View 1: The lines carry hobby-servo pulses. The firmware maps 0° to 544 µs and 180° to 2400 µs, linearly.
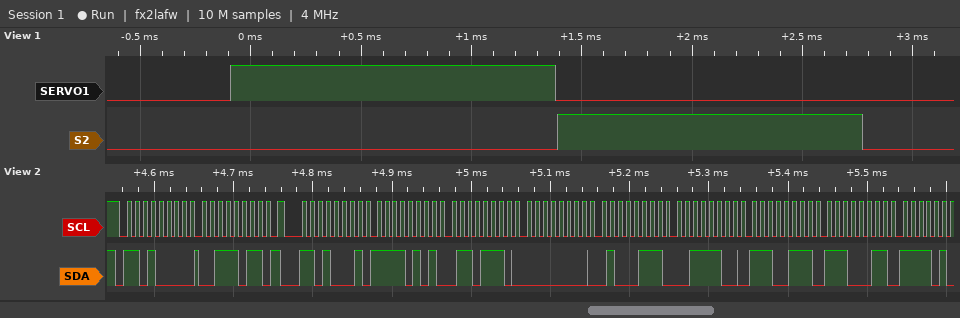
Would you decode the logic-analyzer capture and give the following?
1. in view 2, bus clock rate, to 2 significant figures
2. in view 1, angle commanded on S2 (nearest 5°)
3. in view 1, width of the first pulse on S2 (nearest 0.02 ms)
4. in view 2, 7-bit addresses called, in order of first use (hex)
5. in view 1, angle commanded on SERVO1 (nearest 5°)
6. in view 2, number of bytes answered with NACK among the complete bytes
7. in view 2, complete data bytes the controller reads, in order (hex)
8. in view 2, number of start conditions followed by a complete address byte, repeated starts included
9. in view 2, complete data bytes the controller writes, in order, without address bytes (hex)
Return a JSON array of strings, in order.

["100 kHz", "80°", "1.38 ms", "0x68", "90°", "0", "F5 6E 00 47 3C E7 E3", "2", "3B"]
